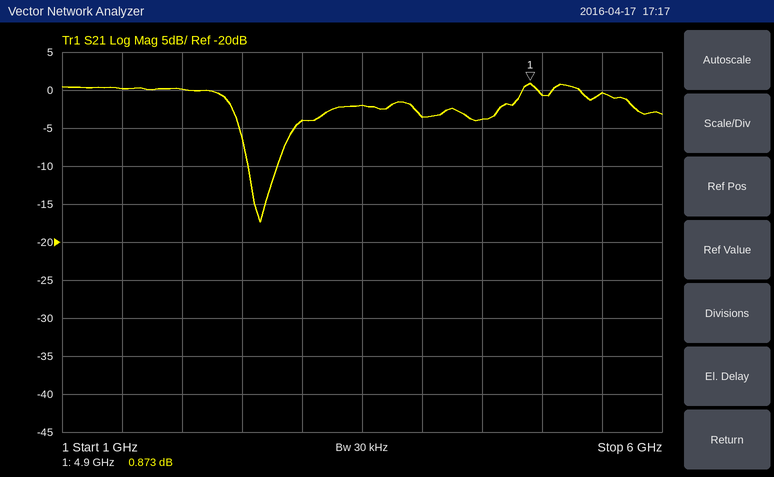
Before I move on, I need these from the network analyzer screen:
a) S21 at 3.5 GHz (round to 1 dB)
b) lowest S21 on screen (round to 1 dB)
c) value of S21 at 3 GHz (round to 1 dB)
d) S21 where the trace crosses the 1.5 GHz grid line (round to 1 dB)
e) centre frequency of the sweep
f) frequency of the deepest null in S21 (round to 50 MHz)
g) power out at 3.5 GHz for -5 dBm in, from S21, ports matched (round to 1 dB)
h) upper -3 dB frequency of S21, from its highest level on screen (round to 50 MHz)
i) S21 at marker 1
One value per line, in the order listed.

-2 dB
-17 dB
-4 dB
0 dB
3.5 GHz
2.65 GHz
-7 dBm
5.75 GHz
0.873 dB
